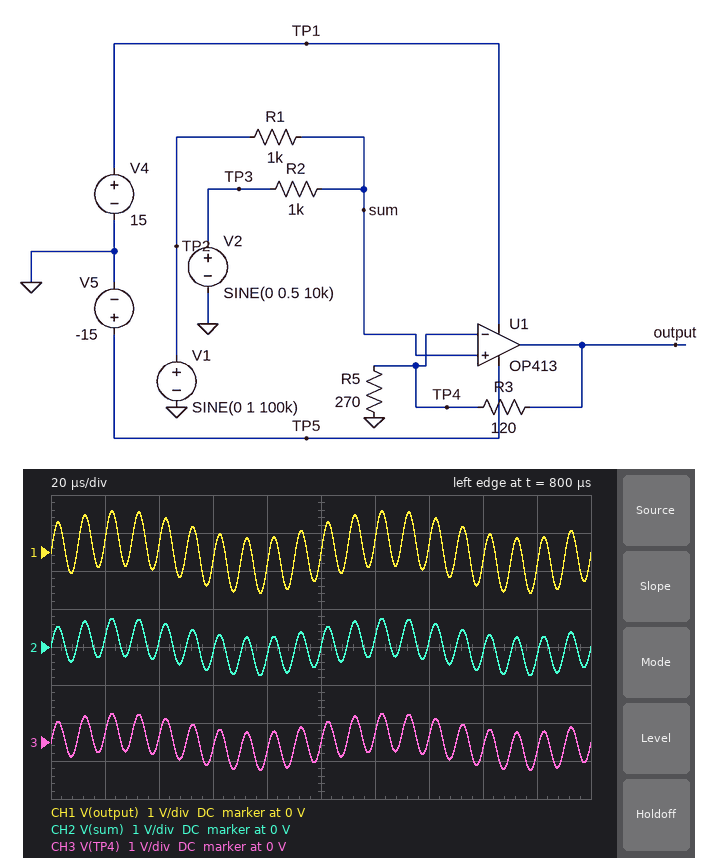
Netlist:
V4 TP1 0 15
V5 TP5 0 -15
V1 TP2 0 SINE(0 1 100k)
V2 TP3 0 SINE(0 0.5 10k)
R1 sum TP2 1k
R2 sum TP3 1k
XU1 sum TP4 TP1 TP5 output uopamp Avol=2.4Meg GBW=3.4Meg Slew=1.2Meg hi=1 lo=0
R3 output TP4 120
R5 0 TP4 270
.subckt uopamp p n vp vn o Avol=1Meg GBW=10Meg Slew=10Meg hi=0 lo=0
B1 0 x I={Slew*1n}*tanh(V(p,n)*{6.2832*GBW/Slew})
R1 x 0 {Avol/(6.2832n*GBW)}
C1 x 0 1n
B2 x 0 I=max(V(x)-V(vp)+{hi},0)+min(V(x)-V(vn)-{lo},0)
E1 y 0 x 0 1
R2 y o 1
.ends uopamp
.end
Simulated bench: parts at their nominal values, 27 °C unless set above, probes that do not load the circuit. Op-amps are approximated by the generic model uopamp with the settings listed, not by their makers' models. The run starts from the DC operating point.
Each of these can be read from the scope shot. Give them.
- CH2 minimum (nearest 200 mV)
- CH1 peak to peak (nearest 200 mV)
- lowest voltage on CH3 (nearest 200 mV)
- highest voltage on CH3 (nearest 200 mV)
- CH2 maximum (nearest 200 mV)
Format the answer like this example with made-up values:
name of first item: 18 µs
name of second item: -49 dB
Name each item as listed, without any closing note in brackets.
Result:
CH2 minimum: -800 mV
CH1 peak to peak: 2.2 V
lowest voltage on CH3: -800 mV
highest voltage on CH3: 800 mV
CH2 maximum: 800 mV
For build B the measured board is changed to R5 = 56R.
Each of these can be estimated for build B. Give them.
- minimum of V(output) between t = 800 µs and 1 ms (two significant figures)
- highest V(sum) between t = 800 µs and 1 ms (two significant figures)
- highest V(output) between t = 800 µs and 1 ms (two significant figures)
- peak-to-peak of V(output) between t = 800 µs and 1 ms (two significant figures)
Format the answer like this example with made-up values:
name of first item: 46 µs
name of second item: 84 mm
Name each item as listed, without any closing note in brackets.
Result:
minimum of V(output) between t = 800 µs and 1 ms: -2.3 V
highest V(sum) between t = 800 µs and 1 ms: 750 mV
highest V(output) between t = 800 µs and 1 ms: 2.3 V
peak-to-peak of V(output) between t = 800 µs and 1 ms: 4.7 V
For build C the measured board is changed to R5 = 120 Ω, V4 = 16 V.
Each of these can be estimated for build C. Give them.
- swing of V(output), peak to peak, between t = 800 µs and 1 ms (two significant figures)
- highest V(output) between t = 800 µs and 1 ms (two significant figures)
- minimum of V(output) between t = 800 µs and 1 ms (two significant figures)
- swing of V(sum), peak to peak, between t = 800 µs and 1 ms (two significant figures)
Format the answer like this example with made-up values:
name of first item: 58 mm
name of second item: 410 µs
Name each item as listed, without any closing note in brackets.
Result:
swing of V(output), peak to peak, between t = 800 µs and 1 ms: 3.0 V
highest V(output) between t = 800 µs and 1 ms: 1.5 V
minimum of V(output) between t = 800 µs and 1 ms: -1.5 V
swing of V(sum), peak to peak, between t = 800 µs and 1 ms: 1.5 V
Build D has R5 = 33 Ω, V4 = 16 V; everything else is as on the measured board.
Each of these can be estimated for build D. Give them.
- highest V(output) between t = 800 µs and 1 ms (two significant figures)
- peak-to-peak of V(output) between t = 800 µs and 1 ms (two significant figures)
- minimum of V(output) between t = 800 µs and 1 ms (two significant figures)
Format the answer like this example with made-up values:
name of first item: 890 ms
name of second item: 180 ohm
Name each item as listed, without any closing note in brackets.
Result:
highest V(output) between t = 800 µs and 1 ms: 3.4 V
peak-to-peak of V(output) between t = 800 µs and 1 ms: 6.8 V
minimum of V(output) between t = 800 µs and 1 ms: -3.4 V
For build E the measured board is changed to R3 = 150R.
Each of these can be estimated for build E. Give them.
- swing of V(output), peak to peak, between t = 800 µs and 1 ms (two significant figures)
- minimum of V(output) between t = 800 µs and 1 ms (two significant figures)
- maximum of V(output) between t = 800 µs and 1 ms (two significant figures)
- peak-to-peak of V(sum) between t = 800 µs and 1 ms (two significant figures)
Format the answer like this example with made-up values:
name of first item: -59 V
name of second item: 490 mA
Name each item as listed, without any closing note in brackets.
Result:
swing of V(output), peak to peak, between t = 800 µs and 1 ms: 2.3 V
minimum of V(output) between t = 800 µs and 1 ms: -1.2 V
maximum of V(output) between t = 800 µs and 1 ms: 1.2 V
peak-to-peak of V(sum) between t = 800 µs and 1 ms: 1.5 V
